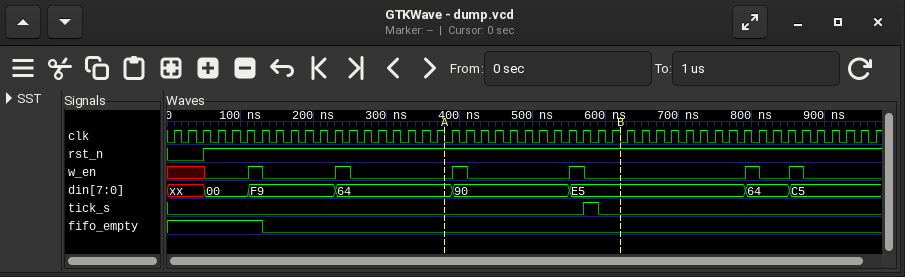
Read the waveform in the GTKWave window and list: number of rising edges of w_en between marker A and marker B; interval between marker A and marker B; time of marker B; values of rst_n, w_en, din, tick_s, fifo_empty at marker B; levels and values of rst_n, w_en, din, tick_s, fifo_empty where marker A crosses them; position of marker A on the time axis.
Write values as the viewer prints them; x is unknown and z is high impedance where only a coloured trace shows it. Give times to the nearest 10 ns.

2
240 ns
620 ns
rst_n=1, w_en=0, din=E5, tick_s=0, fifo_empty=0
rst_n=1, w_en=0, din=64, tick_s=0, fifo_empty=0
380 ns
